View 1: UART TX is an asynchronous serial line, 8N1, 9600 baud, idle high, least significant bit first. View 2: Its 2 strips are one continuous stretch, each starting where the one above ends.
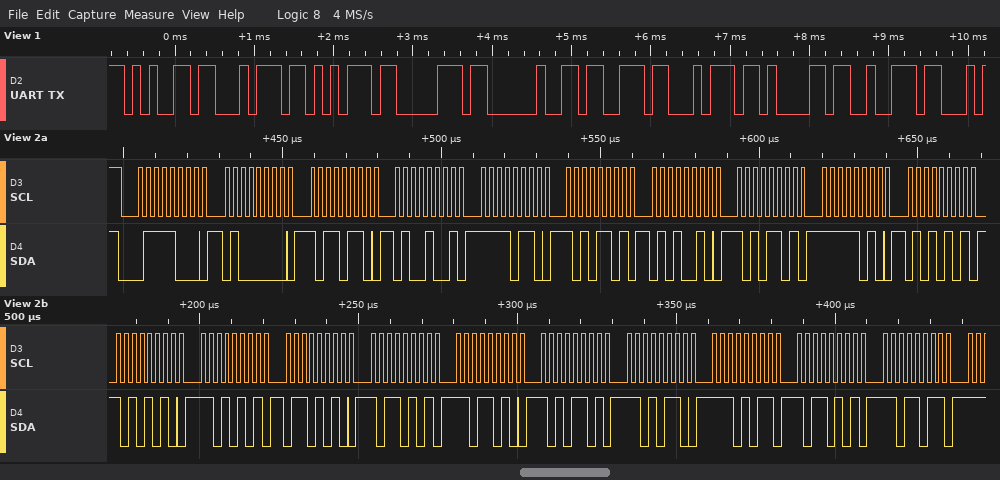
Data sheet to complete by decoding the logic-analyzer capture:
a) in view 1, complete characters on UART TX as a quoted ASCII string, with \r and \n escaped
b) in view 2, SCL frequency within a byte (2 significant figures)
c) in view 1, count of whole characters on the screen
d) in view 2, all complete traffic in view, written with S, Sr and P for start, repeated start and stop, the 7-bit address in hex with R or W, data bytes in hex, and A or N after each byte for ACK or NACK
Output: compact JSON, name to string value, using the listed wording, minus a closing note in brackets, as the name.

{"in view 1, complete characters on UART TX as a quoted ASCII string, with \\r and \\n escaped": "\"etup star\"", "in view 2, SCL frequency within a byte": "400 kHz", "in view 1, count of whole characters on the screen": "9", "in view 2, all complete traffic in view, written with S, Sr and P for start, repeated start and stop, the 7-bit address in hex with R or W, data bytes in hex, and A or N after each byte for ACK or NACK": "S 3CW A 40 A B6 A 49 A F6 A AD A 52 A AD A FA A 55 A AA A D5 A 6A A B5 A DA A AD A D6 A EB A B5 A DB A"}
